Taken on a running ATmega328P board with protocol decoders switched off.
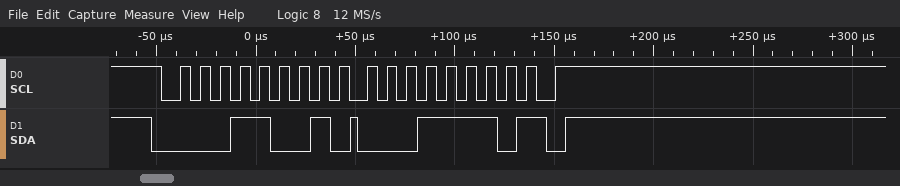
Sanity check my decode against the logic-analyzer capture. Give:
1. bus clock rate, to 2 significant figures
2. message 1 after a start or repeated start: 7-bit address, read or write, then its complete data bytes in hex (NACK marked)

100 kHz
0x0C read: 1E NACK
